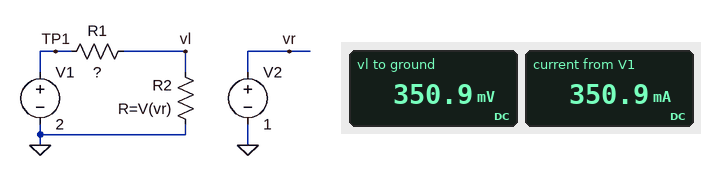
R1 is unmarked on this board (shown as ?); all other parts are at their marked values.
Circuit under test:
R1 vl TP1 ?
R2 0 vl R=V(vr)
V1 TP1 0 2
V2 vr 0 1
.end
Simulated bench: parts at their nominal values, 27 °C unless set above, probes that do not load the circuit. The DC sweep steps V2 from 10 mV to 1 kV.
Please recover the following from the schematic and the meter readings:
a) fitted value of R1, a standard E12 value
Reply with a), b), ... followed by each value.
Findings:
a) 4.7 Ω
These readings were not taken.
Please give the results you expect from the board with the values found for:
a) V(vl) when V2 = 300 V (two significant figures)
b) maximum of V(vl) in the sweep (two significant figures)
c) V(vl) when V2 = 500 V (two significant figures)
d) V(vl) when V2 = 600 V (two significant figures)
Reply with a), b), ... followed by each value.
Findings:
a) 2.0 V
b) 2.0 V
c) 2.0 V
d) 2.0 V
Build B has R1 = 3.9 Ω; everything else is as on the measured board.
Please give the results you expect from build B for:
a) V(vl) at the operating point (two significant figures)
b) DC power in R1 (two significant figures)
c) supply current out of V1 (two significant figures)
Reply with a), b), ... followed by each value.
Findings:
a) 410 mV
b) 650 mW
c) 410 mA
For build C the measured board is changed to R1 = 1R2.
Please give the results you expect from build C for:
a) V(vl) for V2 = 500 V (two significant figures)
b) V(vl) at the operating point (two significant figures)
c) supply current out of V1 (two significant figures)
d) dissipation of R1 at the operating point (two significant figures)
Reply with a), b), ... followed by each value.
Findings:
a) 2.0 V
b) 910 mV
c) 910 mA
d) 990 mW
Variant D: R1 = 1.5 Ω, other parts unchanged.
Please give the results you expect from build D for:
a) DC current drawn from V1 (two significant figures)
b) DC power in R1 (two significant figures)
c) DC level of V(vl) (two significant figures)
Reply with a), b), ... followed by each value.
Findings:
a) 800 mA
b) 960 mW
c) 800 mV
